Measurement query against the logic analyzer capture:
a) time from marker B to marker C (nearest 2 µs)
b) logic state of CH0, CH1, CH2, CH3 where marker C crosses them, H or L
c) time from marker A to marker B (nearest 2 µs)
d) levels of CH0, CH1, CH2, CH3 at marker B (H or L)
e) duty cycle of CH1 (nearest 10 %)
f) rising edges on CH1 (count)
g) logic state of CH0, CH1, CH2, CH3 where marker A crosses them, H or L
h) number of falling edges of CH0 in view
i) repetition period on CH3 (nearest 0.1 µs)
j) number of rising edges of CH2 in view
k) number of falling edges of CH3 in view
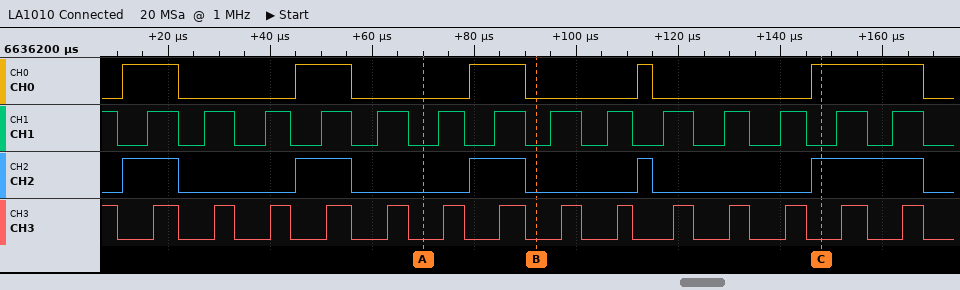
56 µs
CH0=H, CH1=L, CH2=H, CH3=L
22 µs
CH0=L, CH1=L, CH2=L, CH3=L
50 %
14
CH0=L, CH1=L, CH2=L, CH3=L
5
11.3 µs
5
15
